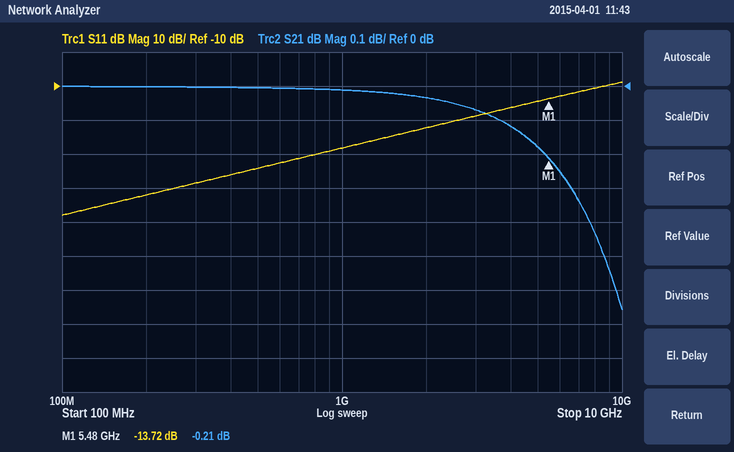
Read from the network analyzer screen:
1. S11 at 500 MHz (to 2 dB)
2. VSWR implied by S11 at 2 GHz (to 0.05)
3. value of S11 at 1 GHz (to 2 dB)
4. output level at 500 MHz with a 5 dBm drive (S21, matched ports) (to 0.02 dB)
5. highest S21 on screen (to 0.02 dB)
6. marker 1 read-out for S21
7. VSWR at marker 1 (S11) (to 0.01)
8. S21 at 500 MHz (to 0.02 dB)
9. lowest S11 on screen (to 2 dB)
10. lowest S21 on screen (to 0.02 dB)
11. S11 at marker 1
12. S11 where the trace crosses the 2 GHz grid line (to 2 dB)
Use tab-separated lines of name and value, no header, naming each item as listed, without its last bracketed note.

S11 at 500 MHz	-34 dB
VSWR implied by S11 at 2 GHz	1.15
value of S11 at 1 GHz	-28 dB
output level at 500 MHz with a 5 dBm drive (S21, matched ports)	5.00 dBm
highest S21 on screen	0.00 dB
marker 1 read-out for S21	-0.21 dB
VSWR at marker 1 (S11)	1.52
S21 at 500 MHz	0.00 dB
lowest S11 on screen	-48 dB
lowest S21 on screen	-0.66 dB
S11 at marker 1	-13.72 dB
S11 where the trace crosses the 2 GHz grid line	-22 dB
